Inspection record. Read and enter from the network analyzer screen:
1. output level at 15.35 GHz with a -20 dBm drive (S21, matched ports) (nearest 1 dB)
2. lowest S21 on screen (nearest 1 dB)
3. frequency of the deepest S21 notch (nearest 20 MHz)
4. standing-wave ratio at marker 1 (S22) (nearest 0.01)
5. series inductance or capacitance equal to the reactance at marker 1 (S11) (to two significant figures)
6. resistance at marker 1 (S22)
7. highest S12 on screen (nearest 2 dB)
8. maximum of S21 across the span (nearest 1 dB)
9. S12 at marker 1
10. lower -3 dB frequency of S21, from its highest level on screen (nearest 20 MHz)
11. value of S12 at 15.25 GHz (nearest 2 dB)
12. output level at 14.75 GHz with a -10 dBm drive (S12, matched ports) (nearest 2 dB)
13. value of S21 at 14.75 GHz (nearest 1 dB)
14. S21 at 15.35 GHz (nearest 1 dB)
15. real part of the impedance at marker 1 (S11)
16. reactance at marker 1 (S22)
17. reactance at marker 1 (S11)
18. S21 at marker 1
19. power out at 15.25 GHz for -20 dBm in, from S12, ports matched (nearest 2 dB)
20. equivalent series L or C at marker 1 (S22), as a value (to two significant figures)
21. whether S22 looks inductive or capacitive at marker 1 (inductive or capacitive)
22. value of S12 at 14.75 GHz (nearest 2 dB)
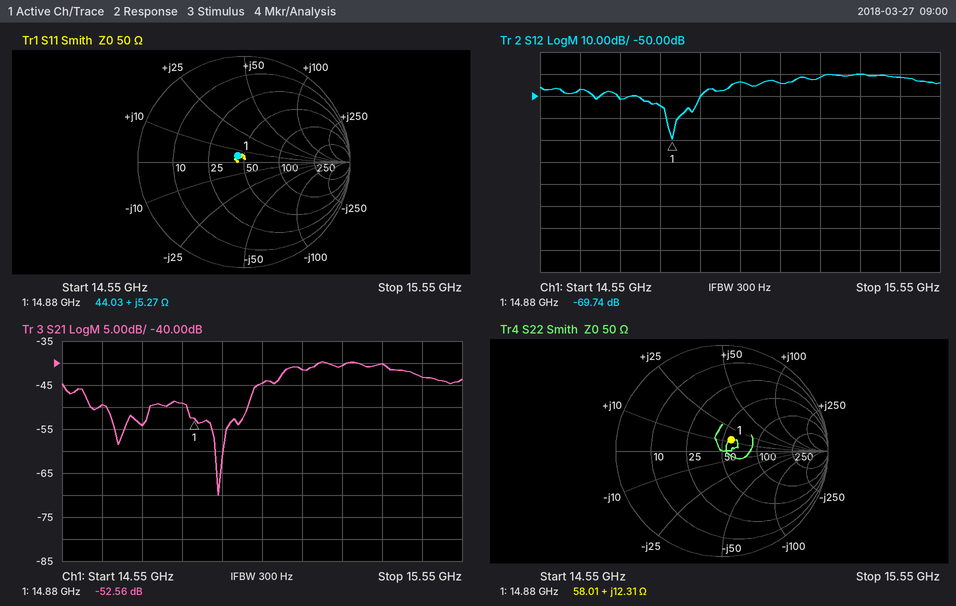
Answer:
-60 dBm
-70 dB
14.94 GHz
1.31
56 pH
58.01 Ω
-40 dB
-40 dB
-69.74 dB
15.10 GHz
-42 dB
-62 dBm
-54 dB
-40 dB
44.03 Ω
+12.31 Ω
+5.27 Ω
-52.56 dB
-62 dBm
130 pH
inductive
-52 dB
